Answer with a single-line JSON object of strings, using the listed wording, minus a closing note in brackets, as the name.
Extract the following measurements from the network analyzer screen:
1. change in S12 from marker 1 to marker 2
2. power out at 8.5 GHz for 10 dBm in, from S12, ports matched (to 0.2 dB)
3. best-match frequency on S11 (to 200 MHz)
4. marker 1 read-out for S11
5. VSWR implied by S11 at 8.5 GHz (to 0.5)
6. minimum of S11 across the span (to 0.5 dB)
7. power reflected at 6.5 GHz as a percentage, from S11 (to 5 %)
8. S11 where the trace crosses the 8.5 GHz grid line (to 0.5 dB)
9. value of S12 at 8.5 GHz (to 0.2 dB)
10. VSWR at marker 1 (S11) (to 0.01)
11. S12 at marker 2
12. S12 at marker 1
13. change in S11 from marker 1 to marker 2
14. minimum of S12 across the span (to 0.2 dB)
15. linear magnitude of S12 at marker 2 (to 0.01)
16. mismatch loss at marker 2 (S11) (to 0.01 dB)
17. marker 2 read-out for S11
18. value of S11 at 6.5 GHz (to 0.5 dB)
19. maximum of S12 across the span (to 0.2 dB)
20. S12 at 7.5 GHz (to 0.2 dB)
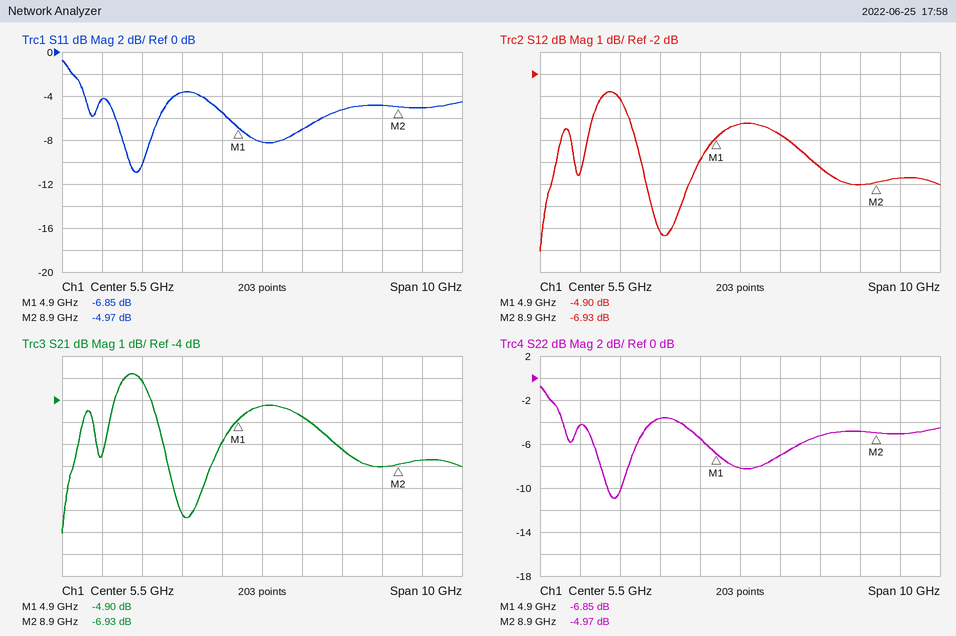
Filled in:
{"change in S12 from marker 1 to marker 2": "-2.03 dB", "power out at 8.5 GHz for 10 dBm in, from S12, ports matched": "3.0 dBm", "best-match frequency on S11": "2.4 GHz", "marker 1 read-out for S11": "-6.85 dB", "VSWR implied by S11 at 8.5 GHz": "3.5", "minimum of S11 across the span": "-11.0 dB", "power reflected at 6.5 GHz as a percentage, from S11": "20 %", "S11 where the trace crosses the 8.5 GHz grid line": "-5.0 dB", "value of S12 at 8.5 GHz": "-7.0 dB", "VSWR at marker 1 (S11)": "2.67", "S12 at marker 2": "-6.93 dB", "S12 at marker 1": "-4.90 dB", "change in S11 from marker 1 to marker 2": "1.88 dB", "minimum of S12 across the span": "-10.0 dB", "linear magnitude of S12 at marker 2": "0.45", "mismatch loss at marker 2 (S11)": "1.66 dB", "marker 2 read-out for S11": "-4.97 dB", "value of S11 at 6.5 GHz": "-7.0 dB", "maximum of S12 across the span": "-2.8 dB", "S12 at 7.5 GHz": "-6.2 dB"}
